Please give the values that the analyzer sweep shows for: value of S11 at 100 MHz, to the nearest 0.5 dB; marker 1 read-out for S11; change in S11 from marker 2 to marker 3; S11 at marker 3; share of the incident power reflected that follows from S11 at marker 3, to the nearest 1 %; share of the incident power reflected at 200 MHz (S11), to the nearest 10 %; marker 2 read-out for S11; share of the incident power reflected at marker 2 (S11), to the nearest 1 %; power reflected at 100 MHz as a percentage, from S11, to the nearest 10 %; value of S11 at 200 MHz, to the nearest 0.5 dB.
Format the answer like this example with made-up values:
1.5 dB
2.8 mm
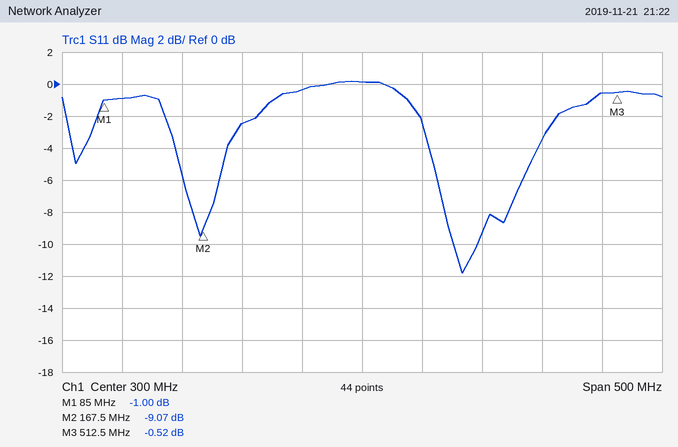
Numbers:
-1.0 dB
-1.00 dB
8.55 dB
-0.52 dB
89 %
60 %
-9.07 dB
12 %
80 %
-2.5 dB
